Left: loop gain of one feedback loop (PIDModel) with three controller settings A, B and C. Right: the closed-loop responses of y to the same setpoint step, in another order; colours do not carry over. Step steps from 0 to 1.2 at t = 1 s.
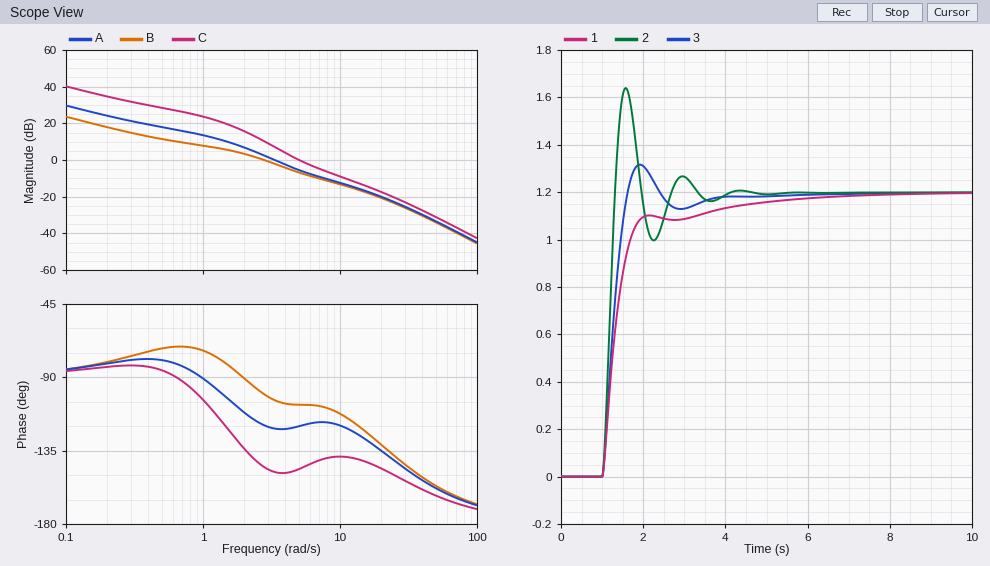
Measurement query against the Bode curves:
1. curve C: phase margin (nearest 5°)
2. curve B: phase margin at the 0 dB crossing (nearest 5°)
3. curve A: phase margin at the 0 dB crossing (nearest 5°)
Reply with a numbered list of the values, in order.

1. 35°
2. 80°
3. 60°
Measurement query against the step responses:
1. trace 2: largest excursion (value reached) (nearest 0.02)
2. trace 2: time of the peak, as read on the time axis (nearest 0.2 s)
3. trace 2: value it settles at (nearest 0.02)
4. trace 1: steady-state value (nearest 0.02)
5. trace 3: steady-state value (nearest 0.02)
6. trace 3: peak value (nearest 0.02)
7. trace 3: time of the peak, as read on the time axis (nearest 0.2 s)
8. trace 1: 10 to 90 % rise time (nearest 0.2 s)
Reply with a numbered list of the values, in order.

1. 1.64
2. 1.6 s
3. 1.20
4. 1.20
5. 1.20
6. 1.32
7. 2.0 s
8. 0.8 s
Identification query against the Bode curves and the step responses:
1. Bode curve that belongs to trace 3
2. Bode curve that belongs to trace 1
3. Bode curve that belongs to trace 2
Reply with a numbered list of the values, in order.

1. A
2. B
3. C
